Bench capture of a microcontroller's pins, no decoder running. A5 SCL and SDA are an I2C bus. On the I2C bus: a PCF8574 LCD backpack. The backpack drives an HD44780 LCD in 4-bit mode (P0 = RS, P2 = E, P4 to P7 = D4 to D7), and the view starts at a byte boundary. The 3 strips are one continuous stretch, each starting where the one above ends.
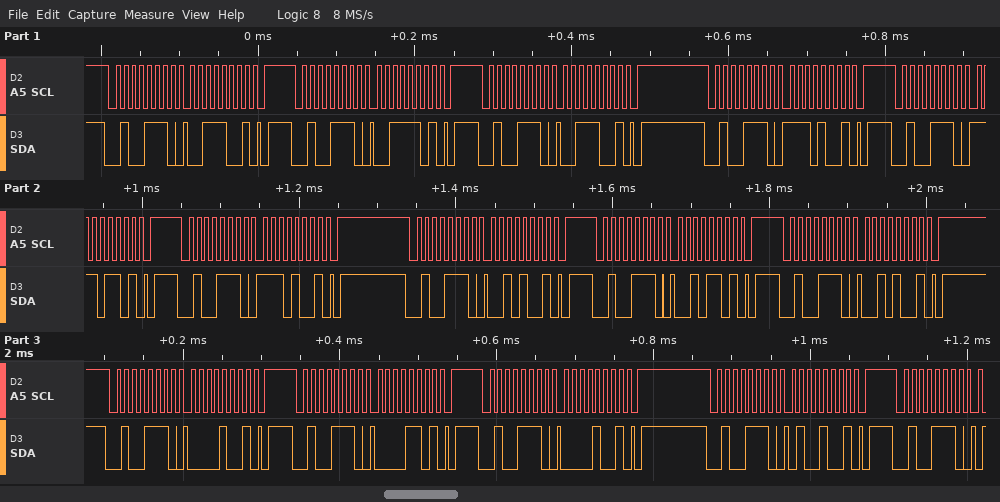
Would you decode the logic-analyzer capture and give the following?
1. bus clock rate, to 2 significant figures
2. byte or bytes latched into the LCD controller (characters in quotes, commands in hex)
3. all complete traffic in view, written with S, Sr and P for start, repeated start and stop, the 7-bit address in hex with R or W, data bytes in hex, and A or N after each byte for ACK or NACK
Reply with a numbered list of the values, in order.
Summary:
1. 100 kHz
2. '>' ' '
3. S 27W A 39 A P S 27W A 3D A P S 27W A 39 A P S 27W A E9 A P S 27W A ED A P S 27W A E9 A P S 27W A 29 A P S 27W A 2D A P S 27W A 29 A P S 27W A 09 A P S 27W A 0D A P S 27W A 09 A P S 27W A 49 A P S 27W A
